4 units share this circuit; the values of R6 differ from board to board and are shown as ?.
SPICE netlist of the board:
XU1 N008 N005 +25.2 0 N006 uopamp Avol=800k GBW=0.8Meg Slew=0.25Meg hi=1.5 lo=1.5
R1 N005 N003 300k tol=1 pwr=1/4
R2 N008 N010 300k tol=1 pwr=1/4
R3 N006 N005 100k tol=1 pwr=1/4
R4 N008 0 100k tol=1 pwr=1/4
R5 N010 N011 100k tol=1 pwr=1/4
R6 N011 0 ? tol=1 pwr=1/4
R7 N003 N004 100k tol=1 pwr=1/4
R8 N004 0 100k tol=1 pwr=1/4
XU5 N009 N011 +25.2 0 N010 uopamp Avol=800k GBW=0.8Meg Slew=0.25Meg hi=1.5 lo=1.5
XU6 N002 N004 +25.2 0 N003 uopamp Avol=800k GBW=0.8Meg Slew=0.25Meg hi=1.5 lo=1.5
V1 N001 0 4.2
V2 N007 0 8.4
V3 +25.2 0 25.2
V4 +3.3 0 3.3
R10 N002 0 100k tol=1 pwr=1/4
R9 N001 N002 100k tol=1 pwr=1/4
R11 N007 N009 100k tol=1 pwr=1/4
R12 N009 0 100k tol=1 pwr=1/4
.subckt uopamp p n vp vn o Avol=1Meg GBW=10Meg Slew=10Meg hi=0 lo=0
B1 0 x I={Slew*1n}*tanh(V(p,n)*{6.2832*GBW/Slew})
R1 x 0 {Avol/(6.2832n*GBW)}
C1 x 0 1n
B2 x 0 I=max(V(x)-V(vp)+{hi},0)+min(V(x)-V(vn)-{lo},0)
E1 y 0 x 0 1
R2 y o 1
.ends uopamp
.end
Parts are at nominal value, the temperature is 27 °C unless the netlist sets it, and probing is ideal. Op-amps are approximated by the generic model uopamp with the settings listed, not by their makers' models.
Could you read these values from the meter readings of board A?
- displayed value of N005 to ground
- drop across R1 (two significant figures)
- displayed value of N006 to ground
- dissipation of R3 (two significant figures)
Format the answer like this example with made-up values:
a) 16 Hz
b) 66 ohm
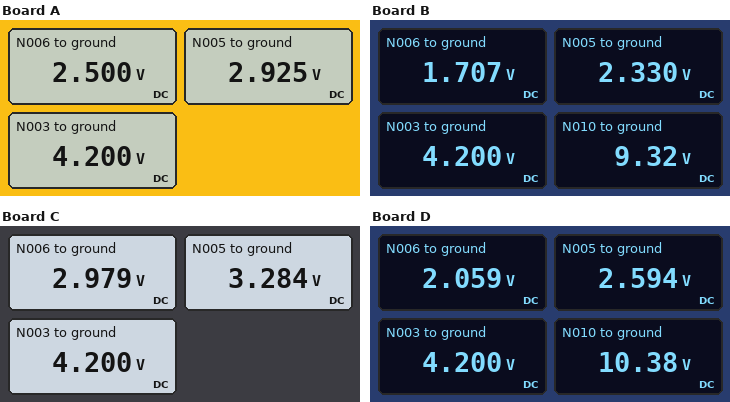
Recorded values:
a) 2.925 V
b) 1.3 V
c) 2.500 V
d) 1.8 µW
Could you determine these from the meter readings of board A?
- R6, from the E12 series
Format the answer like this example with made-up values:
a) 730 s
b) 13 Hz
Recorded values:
a) 56 kΩ
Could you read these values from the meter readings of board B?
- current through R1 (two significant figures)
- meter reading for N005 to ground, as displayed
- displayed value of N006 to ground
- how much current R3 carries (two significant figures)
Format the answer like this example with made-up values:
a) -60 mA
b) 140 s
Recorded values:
a) 6.2 µA
b) 2.330 V
c) 1.707 V
d) 6.2 µA
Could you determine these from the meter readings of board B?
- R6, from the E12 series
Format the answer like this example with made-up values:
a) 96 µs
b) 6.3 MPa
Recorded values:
a) 82 kΩ
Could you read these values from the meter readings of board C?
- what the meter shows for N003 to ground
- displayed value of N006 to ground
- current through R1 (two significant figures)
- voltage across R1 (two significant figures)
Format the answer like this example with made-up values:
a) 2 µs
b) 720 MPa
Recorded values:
a) 4.200 V
b) 2.979 V
c) 3.1 µA
d) 920 mV
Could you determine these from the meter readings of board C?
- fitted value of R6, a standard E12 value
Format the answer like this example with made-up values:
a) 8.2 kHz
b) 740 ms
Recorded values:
a) 47 kΩ
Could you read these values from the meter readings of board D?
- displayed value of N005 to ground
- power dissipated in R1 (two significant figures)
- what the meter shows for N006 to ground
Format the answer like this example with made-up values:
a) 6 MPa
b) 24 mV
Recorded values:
a) 2.594 V
b) 8.6 µW
c) 2.059 V
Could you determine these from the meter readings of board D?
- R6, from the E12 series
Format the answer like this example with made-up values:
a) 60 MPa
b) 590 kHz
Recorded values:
a) 68 kΩ
